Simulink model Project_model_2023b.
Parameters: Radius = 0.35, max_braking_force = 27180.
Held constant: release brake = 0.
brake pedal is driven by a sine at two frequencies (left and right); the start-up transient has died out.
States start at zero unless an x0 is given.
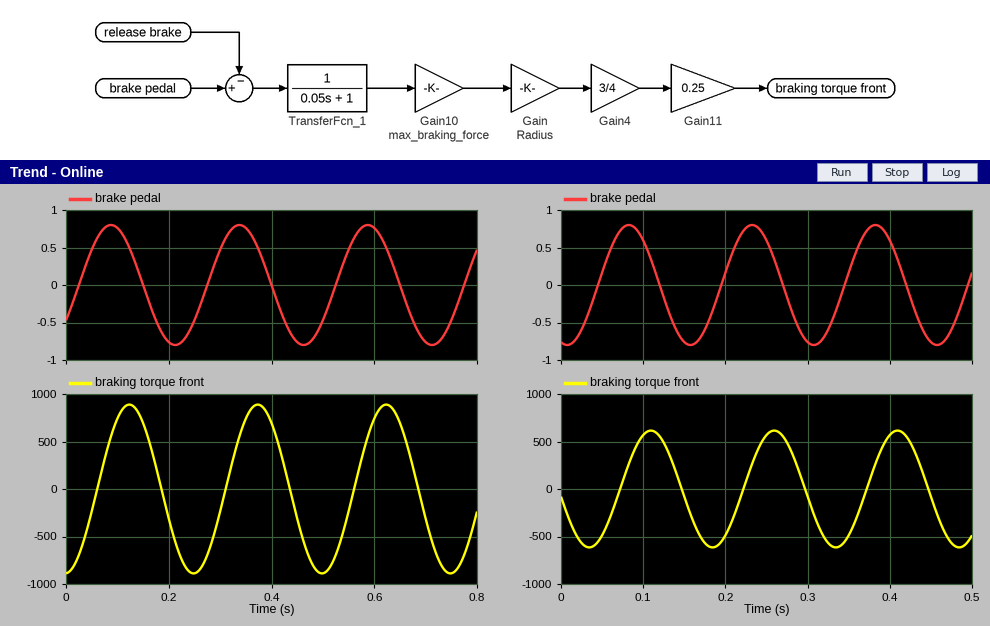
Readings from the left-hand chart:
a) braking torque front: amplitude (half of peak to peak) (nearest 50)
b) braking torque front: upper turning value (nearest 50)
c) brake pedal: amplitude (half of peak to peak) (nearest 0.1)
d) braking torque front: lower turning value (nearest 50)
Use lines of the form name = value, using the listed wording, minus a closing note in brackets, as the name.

braking torque front: amplitude (half of peak to peak) = 900
braking torque front: upper turning value = 900
brake pedal: amplitude (half of peak to peak) = 0.8
braking torque front: lower turning value = -900
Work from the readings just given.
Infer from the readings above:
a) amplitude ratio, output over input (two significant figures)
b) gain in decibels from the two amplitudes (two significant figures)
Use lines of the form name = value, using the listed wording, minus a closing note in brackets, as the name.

amplitude ratio, output over input = 1100
gain in decibels from the two amplitudes = 61 dB
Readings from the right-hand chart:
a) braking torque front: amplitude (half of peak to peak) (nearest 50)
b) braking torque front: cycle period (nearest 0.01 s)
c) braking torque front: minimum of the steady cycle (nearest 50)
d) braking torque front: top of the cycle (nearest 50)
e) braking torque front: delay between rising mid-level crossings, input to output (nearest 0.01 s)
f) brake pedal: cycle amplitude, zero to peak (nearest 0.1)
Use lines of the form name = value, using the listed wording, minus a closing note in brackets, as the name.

braking torque front: amplitude (half of peak to peak) = 600
braking torque front: cycle period = 0.15 s
braking torque front: minimum of the steady cycle = -600
braking torque front: top of the cycle = 600
braking torque front: delay between rising mid-level crossings, input to output = 0.03 s
brake pedal: cycle amplitude, zero to peak = 0.8
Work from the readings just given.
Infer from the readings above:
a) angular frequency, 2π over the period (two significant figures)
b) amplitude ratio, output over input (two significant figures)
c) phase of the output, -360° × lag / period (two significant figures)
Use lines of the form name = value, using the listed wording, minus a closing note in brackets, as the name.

angular frequency, 2π over the period = 42 rad/s
amplitude ratio, output over input = 750
phase of the output, -360° × lag / period = -72°
